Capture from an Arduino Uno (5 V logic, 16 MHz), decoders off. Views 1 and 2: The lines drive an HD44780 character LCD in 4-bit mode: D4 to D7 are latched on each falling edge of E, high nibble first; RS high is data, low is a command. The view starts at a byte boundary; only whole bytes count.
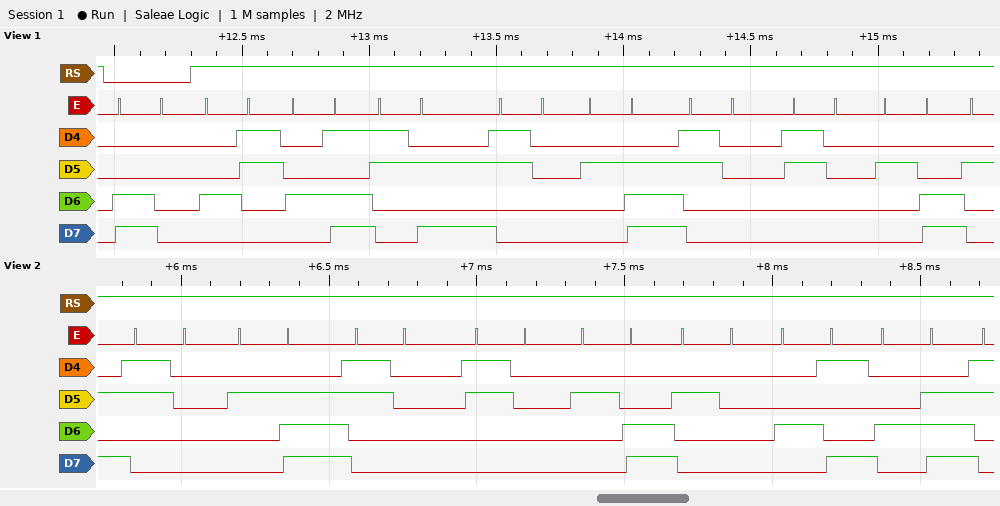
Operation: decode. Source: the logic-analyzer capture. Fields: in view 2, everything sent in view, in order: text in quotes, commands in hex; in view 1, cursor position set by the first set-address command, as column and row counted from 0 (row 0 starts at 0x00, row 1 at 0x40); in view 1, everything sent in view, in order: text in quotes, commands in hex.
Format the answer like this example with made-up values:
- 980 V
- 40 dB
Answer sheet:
- "0.00, IN"
- column 0, row 1
- 0xC0 "CM:0.00,"
